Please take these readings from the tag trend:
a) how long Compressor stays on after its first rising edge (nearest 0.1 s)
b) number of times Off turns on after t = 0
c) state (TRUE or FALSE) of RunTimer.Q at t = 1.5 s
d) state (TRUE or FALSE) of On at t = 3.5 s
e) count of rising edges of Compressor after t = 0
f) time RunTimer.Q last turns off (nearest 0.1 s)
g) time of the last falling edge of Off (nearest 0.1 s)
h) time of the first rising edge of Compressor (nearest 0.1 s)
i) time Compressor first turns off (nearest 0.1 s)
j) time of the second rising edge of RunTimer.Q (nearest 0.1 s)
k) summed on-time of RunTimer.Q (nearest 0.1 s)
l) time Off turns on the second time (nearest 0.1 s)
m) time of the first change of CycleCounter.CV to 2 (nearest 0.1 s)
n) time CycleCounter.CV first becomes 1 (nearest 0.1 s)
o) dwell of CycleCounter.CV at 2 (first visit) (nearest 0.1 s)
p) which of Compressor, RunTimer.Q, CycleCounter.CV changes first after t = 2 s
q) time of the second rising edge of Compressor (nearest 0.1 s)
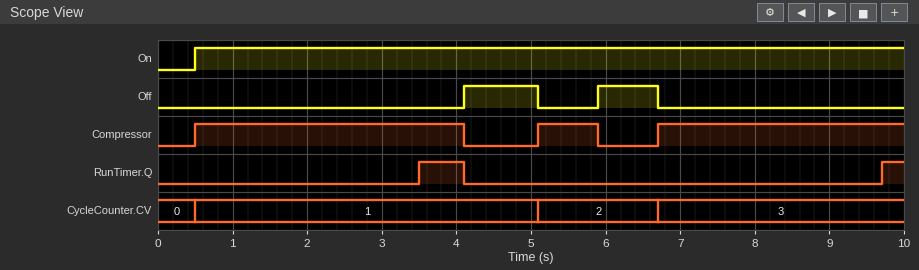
3.6 s
2
FALSE
TRUE
3
4.1 s
6.7 s
0.5 s
4.1 s
9.7 s
0.9 s
5.9 s
5.1 s
0.5 s
1.6 s
RunTimer.Q
5.1 s
